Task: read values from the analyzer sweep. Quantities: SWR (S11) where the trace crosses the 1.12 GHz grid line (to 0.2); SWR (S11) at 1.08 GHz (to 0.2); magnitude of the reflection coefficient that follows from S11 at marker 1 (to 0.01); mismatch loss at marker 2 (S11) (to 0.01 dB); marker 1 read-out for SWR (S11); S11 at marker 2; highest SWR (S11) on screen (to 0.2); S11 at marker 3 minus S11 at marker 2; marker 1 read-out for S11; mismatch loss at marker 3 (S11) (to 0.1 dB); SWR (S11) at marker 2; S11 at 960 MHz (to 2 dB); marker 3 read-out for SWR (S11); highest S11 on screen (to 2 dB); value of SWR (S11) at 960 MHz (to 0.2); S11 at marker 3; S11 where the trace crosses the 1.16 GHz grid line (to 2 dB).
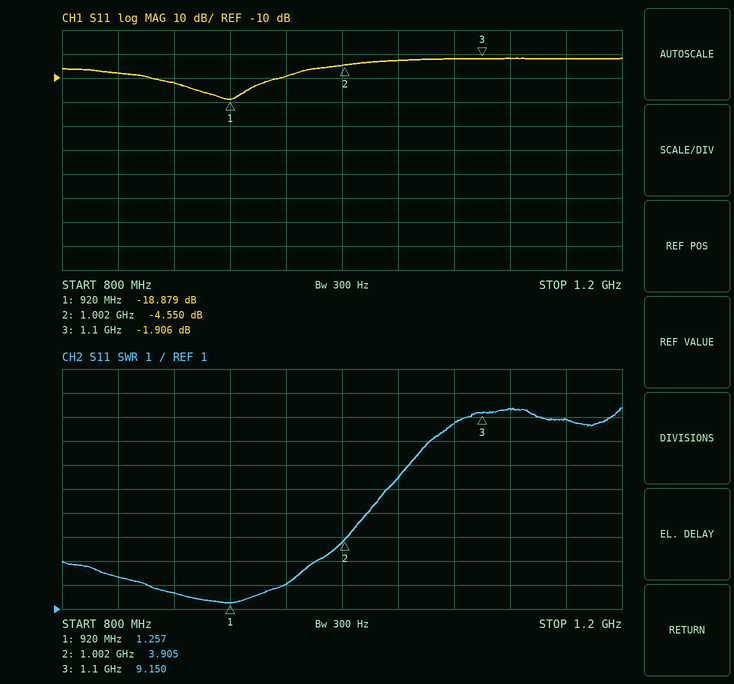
9.4
8.8
0.11
1.88 dB
1.257
-4.550 dB
9.4
2.644 dB
-18.879 dB
4.5 dB
3.905
-10 dB
9.150
-2 dB
2.0
-1.906 dB
-2 dB
